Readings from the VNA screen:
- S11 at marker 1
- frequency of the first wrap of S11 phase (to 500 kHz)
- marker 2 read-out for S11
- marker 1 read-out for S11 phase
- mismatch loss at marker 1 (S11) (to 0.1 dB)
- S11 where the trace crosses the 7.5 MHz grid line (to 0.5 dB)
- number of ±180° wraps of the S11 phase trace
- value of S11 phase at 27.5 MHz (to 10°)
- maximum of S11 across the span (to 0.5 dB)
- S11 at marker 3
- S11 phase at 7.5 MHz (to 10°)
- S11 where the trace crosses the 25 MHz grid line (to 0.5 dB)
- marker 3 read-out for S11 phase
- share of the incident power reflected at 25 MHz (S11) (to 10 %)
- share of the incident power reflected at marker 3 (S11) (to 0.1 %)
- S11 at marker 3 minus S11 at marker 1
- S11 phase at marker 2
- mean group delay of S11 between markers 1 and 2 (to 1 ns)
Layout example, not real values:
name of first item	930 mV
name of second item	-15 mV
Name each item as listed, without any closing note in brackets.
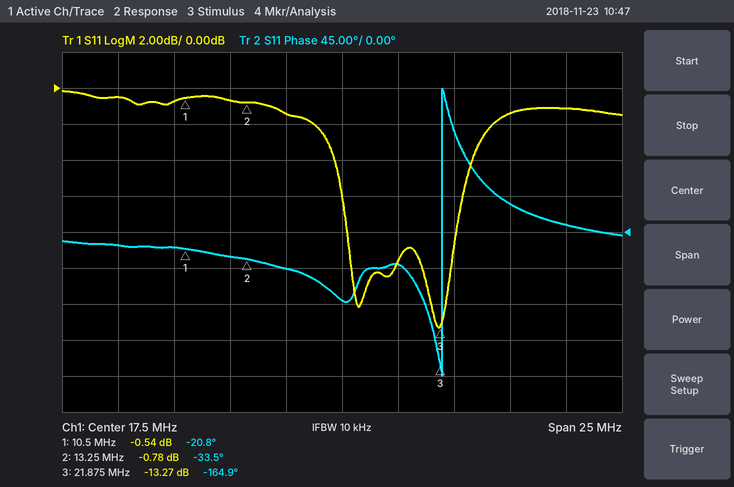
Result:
S11 at marker 1	-0.54 dB
frequency of the first wrap of S11 phase	22.0 MHz
marker 2 read-out for S11	-0.78 dB
marker 1 read-out for S11 phase	-20.8°
mismatch loss at marker 1 (S11)	9.3 dB
S11 where the trace crosses the 7.5 MHz grid line	-0.5 dB
number of ±180° wraps of the S11 phase trace	1
value of S11 phase at 27.5 MHz	10°
maximum of S11 across the span	0.0 dB
S11 at marker 3	-13.27 dB
S11 phase at 7.5 MHz	-20°
S11 where the trace crosses the 25 MHz grid line	-1.5 dB
marker 3 read-out for S11 phase	-164.9°
share of the incident power reflected at 25 MHz (S11)	70 %
share of the incident power reflected at marker 3 (S11)	4.7 %
S11 at marker 3 minus S11 at marker 1	-12.73 dB
S11 phase at marker 2	-33.5°
mean group delay of S11 between markers 1 and 2	13 ns
